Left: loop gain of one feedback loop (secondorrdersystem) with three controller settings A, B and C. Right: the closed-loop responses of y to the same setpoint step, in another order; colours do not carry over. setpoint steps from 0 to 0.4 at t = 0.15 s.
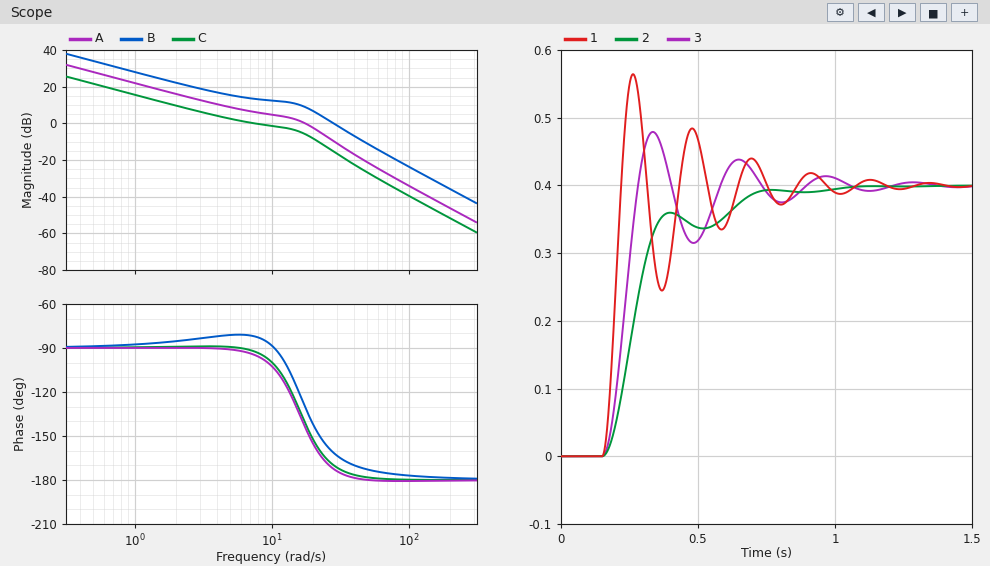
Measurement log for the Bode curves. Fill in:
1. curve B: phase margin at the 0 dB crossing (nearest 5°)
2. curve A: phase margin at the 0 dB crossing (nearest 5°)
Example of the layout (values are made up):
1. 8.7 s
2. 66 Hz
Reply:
1. 20°
2. 35°
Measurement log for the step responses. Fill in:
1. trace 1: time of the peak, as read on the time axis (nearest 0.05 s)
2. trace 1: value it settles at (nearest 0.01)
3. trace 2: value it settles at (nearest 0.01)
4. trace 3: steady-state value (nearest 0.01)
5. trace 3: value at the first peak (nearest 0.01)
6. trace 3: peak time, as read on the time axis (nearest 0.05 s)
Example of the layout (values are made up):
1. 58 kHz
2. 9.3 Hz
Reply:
1. 0.25 s
2. 0.40
3. 0.40
4. 0.40
5. 0.48
6. 0.35 s
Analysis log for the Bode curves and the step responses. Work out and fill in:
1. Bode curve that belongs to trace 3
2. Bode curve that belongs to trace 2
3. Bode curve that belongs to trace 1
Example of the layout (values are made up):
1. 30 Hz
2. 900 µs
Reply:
1. A
2. C
3. B
